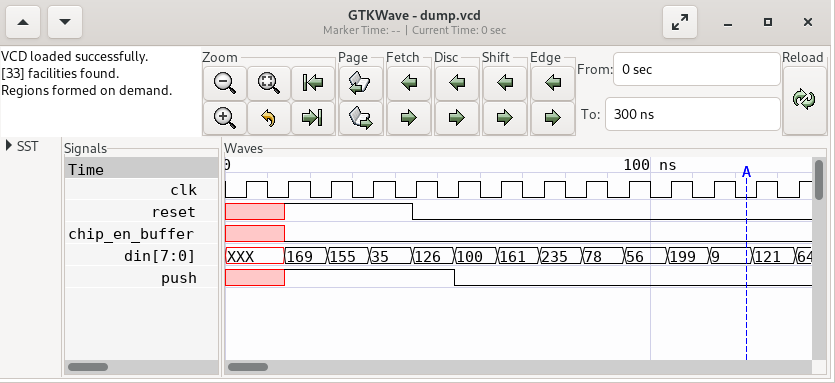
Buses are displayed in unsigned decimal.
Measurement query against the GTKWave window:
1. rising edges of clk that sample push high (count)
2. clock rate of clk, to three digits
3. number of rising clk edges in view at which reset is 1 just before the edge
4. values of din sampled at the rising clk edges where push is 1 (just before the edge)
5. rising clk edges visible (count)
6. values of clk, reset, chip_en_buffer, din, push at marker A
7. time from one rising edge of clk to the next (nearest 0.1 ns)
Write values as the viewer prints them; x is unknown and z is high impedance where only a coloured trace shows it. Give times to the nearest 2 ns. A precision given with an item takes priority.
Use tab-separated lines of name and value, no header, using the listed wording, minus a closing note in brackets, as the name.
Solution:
rising edges of clk that sample push high	4
clock rate of clk, to three digits	100 MHz
number of rising clk edges in view at which reset is 1 just before the edge	3
values of din sampled at the rising clk edges where push is 1	169, 155, 35, 126
rising clk edges visible	14
values of clk, reset, chip_en_buffer, din, push at marker A	clk=0, reset=0, chip_en_buffer=0, din=9, push=0
time from one rising edge of clk to the next	10 ns
